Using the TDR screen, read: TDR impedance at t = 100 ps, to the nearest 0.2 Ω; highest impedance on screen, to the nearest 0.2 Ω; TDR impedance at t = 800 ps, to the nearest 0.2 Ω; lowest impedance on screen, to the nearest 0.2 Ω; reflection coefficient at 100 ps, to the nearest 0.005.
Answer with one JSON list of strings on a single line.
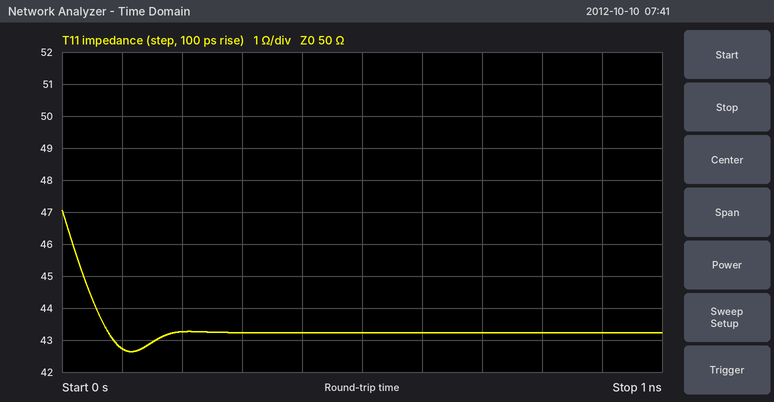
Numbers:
["42.8 Ω", "47.0 Ω", "43.2 Ω", "42.6 Ω", "-0.080"]
